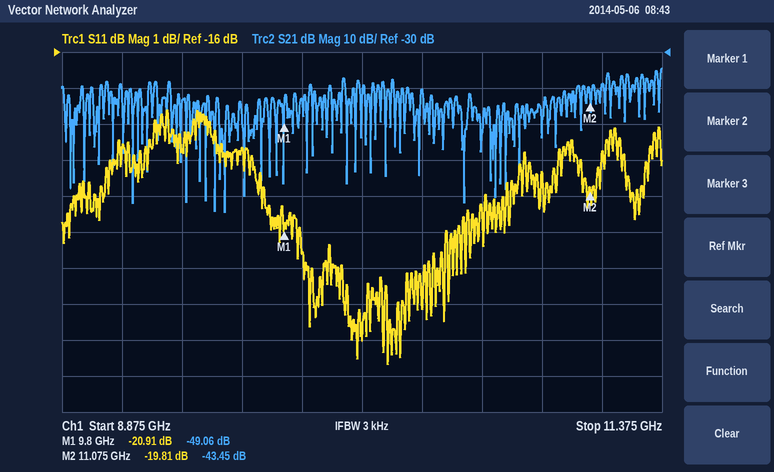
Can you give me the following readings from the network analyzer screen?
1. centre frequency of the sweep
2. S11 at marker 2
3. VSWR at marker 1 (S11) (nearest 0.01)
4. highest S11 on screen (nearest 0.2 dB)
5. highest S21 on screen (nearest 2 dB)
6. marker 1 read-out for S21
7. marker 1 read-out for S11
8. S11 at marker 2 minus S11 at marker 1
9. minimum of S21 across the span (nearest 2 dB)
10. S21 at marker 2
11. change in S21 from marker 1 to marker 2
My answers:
10.125 GHz
-19.81 dB
1.20
-17.6 dB
-34 dB
-49.06 dB
-20.91 dB
1.10 dB
-74 dB
-43.45 dB
5.61 dB
